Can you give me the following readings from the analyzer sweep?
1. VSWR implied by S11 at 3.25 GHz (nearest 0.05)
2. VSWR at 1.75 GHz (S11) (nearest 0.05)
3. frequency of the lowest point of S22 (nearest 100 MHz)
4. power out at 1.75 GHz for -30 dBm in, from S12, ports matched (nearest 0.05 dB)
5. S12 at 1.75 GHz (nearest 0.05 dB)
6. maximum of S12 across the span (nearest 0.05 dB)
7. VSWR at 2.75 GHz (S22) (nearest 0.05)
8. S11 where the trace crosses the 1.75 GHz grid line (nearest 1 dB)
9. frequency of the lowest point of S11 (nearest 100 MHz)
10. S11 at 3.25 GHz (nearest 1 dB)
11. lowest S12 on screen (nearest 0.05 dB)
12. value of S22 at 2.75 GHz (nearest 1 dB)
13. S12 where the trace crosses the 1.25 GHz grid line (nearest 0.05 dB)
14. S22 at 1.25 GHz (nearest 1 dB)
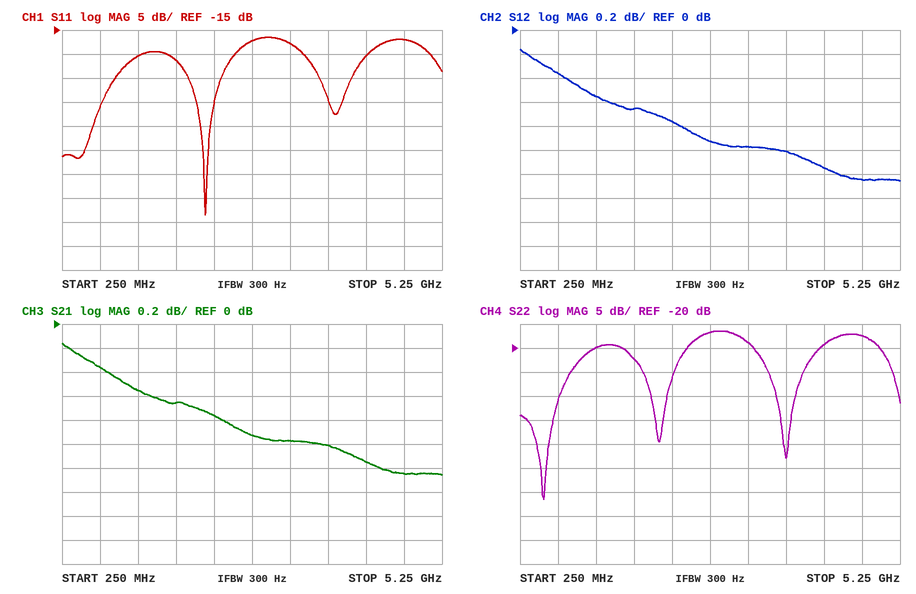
1.30
1.20
600 MHz
-30.65 dBm
-0.65 dB
-0.15 dB
1.35
-21 dB
2.1 GHz
-18 dB
-1.25 dB
-17 dB
-0.55 dB
-20 dB
